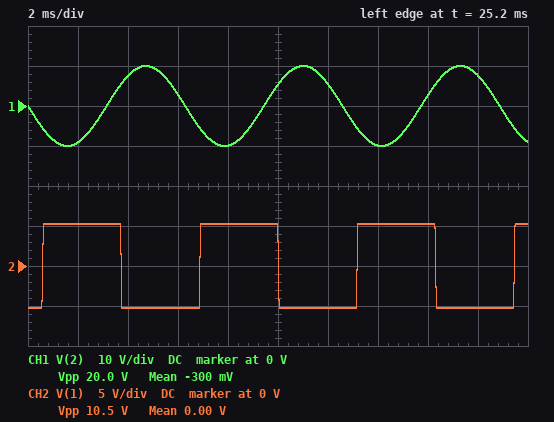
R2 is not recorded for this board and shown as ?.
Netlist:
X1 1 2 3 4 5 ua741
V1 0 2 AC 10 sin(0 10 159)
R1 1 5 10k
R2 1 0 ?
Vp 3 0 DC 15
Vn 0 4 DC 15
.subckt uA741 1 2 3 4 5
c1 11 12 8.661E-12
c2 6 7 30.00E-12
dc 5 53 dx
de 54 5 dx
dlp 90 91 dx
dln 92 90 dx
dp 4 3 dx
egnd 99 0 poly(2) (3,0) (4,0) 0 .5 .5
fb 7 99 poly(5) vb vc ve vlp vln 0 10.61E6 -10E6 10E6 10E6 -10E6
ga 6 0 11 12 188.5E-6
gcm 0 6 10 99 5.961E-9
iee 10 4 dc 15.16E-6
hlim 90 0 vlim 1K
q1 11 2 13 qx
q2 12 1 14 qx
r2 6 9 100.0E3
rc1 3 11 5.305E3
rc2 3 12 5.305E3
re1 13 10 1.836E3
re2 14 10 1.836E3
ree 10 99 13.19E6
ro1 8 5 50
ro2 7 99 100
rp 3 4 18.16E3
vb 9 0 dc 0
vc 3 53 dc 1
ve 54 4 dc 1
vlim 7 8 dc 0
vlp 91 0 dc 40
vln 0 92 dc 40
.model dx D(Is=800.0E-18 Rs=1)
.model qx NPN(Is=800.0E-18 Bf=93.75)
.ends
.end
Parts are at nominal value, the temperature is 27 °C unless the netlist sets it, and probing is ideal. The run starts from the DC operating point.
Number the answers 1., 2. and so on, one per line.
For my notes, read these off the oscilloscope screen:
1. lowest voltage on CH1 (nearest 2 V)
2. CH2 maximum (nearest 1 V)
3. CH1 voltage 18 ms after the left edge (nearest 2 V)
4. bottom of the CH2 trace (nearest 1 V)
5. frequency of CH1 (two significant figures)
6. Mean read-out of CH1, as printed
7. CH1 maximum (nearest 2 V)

1. -10 V
2. 5 V
3. 8 V
4. -5 V
5. 160 Hz
6. -300 mV
7. 10 V
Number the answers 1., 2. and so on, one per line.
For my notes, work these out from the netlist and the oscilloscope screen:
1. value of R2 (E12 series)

1. 5.6 kΩ
